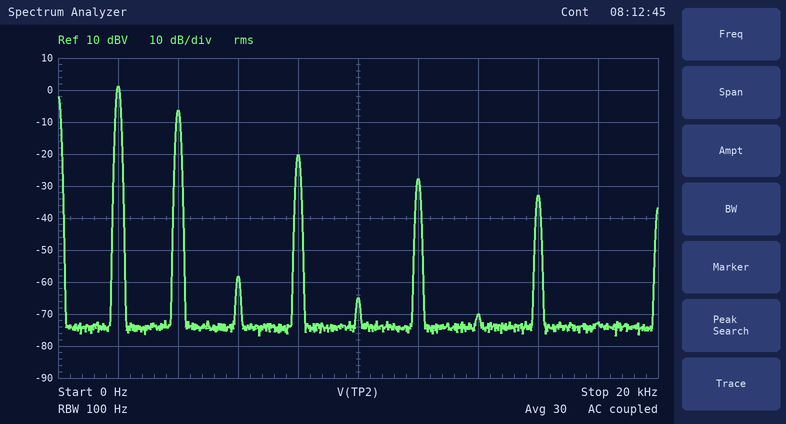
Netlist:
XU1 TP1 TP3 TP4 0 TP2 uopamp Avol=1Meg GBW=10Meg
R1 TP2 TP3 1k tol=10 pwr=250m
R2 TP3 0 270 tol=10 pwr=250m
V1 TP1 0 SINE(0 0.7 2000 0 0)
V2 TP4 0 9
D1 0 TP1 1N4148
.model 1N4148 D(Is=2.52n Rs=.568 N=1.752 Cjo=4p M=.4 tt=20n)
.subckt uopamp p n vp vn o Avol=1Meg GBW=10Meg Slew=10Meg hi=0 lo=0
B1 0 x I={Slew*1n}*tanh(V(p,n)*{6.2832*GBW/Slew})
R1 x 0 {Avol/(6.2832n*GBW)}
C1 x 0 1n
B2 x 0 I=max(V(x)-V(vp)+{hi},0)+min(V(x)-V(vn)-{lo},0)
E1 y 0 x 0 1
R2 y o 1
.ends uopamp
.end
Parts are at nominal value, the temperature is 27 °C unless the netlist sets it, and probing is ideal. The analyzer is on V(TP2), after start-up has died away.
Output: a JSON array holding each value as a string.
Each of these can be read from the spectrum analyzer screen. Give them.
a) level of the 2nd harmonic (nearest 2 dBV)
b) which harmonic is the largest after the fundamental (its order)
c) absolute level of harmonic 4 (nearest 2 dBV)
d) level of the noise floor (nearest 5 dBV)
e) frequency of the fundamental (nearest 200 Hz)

["-6 dBV", "2", "-20 dBV", "-75 dBV", "2.0 kHz"]
